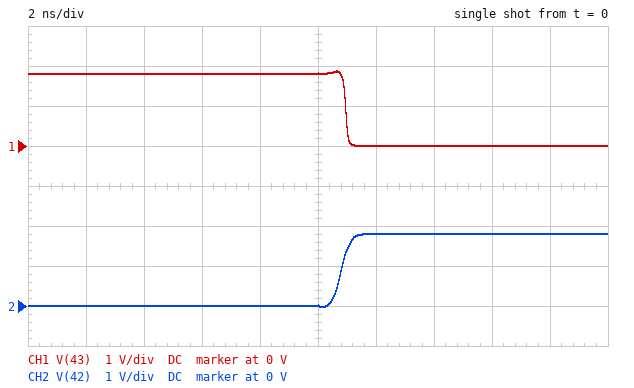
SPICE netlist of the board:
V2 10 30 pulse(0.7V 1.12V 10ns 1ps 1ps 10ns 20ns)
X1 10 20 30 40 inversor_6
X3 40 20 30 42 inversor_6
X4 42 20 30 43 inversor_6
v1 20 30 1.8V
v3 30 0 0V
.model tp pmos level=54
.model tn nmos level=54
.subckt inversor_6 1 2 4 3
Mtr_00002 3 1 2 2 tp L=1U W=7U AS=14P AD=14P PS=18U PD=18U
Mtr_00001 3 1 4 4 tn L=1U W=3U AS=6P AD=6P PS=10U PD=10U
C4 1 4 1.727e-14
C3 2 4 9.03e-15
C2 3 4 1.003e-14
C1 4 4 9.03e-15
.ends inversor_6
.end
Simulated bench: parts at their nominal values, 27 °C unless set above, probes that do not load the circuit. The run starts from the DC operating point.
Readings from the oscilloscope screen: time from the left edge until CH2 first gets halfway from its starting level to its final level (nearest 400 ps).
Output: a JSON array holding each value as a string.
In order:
["10.8 ns"]
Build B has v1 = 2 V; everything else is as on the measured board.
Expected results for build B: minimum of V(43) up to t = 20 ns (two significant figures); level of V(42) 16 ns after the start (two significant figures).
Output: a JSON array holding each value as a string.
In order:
["-22 mV", "2.0 V"]
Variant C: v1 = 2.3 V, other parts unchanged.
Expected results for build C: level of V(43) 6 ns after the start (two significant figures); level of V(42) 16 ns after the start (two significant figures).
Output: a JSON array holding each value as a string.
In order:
["2.3 V", "100 mV"]
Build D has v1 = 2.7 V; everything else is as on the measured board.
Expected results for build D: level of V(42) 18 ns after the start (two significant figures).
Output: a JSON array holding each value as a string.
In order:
["15 mV"]
